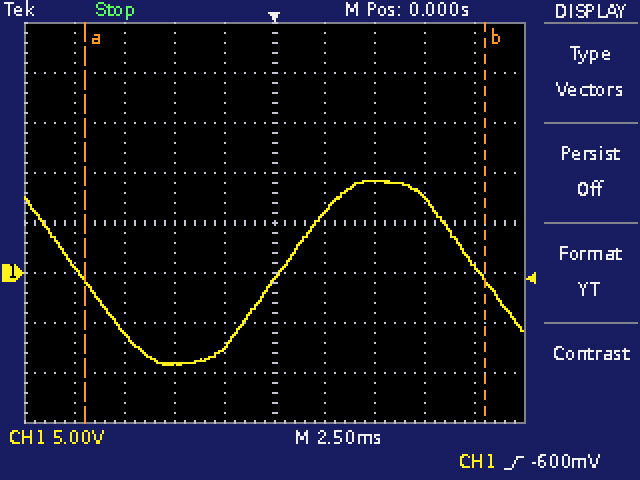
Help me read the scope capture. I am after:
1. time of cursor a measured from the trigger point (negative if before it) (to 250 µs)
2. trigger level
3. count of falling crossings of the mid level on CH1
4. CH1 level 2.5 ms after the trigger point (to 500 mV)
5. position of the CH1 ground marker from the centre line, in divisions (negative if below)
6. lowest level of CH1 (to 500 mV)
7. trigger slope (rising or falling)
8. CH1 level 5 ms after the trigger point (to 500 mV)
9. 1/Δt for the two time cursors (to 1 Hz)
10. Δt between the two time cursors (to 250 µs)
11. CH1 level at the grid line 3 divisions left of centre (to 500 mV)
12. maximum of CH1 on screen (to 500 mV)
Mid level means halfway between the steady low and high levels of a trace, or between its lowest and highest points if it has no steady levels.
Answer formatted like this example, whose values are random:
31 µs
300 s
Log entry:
-9.50 ms
-600 mV
2
6.0 V
-1.0 div
-9.0 V
rising
9.0 V
50 Hz
20.00 ms
-6.0 V
9.0 V
